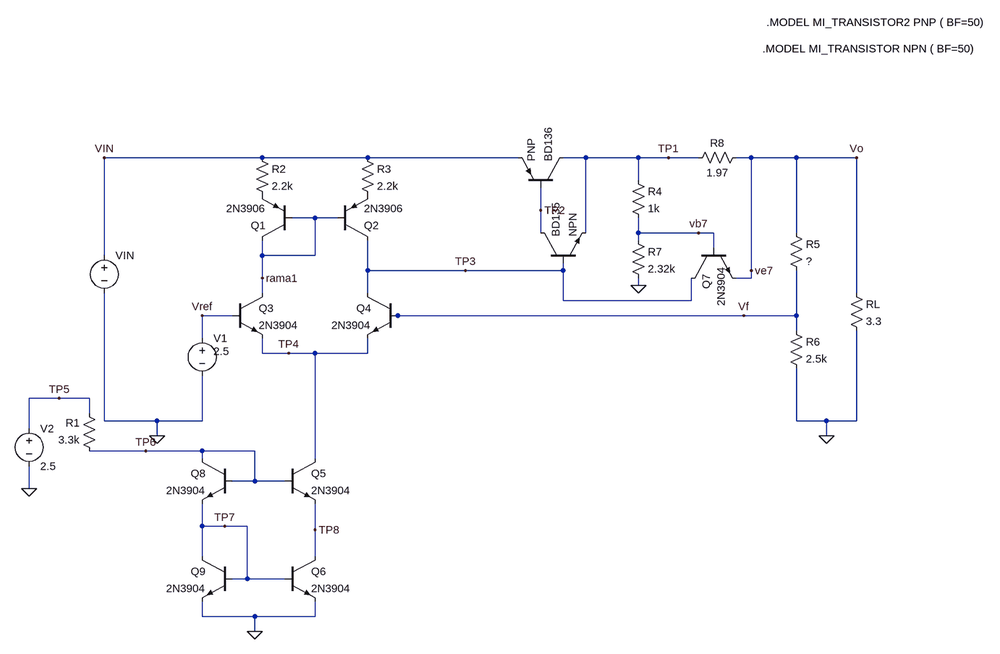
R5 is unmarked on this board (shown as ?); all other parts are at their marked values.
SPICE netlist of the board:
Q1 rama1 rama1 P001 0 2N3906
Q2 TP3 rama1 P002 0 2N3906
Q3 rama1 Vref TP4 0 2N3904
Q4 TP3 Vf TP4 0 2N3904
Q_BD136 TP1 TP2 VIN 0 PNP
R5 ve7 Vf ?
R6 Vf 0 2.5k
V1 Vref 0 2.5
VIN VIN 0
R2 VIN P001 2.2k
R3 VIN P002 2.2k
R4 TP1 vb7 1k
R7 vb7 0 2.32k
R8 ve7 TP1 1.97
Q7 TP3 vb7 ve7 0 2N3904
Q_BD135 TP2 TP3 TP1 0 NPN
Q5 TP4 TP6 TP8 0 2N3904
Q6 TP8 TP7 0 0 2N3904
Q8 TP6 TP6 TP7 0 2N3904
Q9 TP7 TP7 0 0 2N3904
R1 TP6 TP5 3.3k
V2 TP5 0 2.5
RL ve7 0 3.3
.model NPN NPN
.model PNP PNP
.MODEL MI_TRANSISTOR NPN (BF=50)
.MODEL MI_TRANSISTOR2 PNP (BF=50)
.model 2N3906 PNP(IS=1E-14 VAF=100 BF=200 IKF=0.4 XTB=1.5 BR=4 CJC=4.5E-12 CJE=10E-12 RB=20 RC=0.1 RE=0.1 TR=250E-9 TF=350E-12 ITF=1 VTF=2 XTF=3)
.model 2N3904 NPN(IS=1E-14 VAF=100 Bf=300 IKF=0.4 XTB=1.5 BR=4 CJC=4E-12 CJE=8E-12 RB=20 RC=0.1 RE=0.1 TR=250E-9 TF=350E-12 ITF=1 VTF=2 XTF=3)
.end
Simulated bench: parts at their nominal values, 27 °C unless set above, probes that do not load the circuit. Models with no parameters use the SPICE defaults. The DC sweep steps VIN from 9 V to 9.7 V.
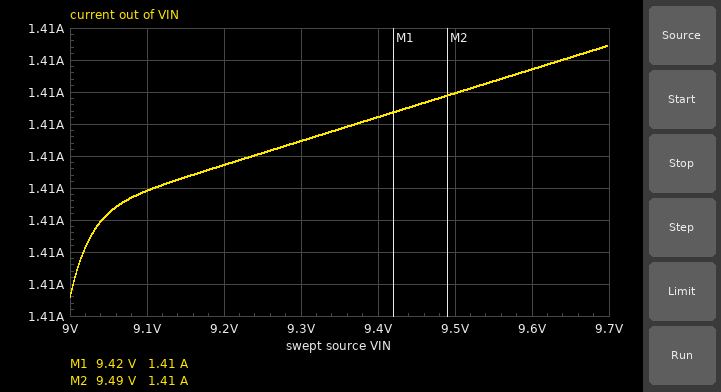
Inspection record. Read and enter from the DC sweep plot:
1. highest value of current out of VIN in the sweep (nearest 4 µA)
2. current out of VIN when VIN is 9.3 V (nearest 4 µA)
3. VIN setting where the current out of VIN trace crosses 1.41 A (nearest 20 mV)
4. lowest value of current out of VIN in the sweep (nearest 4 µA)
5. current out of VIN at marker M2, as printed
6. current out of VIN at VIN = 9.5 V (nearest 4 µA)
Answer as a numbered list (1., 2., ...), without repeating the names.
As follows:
1. 1.414888 A
2. 1.414828 A
3. 9.50 V
4. 1.414732 A
5. 1.41 A
6. 1.414860 A
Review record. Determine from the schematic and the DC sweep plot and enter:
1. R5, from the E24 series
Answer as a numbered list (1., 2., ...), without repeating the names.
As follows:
1. 2.2 kΩ
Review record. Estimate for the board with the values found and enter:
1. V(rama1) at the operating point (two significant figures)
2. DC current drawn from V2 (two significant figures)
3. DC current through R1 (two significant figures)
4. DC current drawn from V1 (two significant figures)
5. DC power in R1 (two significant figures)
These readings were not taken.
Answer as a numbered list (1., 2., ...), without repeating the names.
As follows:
1. 1.8 V
2. 380 µA
3. 380 µA
4. 370 µA
5. 470 µW
